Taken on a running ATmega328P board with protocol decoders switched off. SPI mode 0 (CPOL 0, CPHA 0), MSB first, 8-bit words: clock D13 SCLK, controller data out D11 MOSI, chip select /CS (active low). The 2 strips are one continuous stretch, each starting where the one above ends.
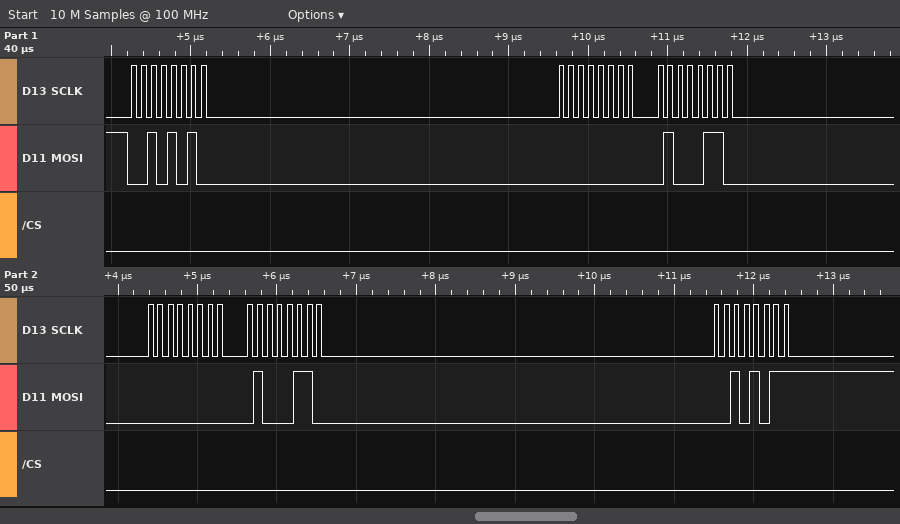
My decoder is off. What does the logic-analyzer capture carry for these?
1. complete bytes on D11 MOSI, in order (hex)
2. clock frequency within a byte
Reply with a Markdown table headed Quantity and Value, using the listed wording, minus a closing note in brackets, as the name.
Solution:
| Quantity | Value |
|---|---|
| complete bytes on D11 MOSI, in order | 2A 00 46 00 46 2B |
| clock frequency within a byte | 8 MHz |
